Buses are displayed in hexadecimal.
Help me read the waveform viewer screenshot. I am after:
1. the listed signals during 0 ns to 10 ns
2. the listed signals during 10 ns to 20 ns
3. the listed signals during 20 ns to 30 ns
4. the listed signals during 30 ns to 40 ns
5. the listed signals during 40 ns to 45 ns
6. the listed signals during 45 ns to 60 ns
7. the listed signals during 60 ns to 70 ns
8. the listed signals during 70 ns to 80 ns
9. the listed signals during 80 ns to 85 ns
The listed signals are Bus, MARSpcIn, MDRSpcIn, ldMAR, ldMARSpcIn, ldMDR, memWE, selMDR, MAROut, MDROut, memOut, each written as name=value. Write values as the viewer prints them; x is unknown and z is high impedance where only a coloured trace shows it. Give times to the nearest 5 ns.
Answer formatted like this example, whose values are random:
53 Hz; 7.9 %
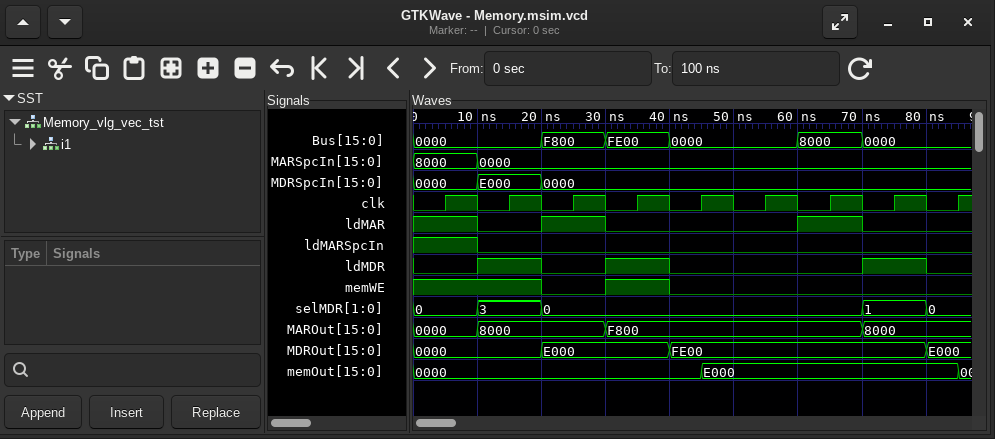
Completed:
Bus=0000, MARSpcIn=8000, MDRSpcIn=0000, ldMAR=1, ldMARSpcIn=1, ldMDR=0, memWE=1, selMDR=0, MAROut=0000, MDROut=0000, memOut=0000; Bus=0000, MARSpcIn=0000, MDRSpcIn=E000, ldMAR=0, ldMARSpcIn=0, ldMDR=1, memWE=1, selMDR=3, MAROut=8000, MDROut=0000, memOut=0000; Bus=F800, MARSpcIn=0000, MDRSpcIn=0000, ldMAR=1, ldMARSpcIn=0, ldMDR=0, memWE=0, selMDR=0, MAROut=8000, MDROut=E000, memOut=0000; Bus=FE00, MARSpcIn=0000, MDRSpcIn=0000, ldMAR=0, ldMARSpcIn=0, ldMDR=1, memWE=1, selMDR=0, MAROut=F800, MDROut=E000, memOut=0000; Bus=0000, MARSpcIn=0000, MDRSpcIn=0000, ldMAR=0, ldMARSpcIn=0, ldMDR=0, memWE=0, selMDR=0, MAROut=F800, MDROut=FE00, memOut=0000; Bus=0000, MARSpcIn=0000, MDRSpcIn=0000, ldMAR=0, ldMARSpcIn=0, ldMDR=0, memWE=0, selMDR=0, MAROut=F800, MDROut=FE00, memOut=E000; Bus=8000, MARSpcIn=0000, MDRSpcIn=0000, ldMAR=1, ldMARSpcIn=0, ldMDR=0, memWE=0, selMDR=0, MAROut=F800, MDROut=FE00, memOut=E000; Bus=0000, MARSpcIn=0000, MDRSpcIn=0000, ldMAR=0, ldMARSpcIn=0, ldMDR=1, memWE=0, selMDR=1, MAROut=8000, MDROut=FE00, memOut=E000; Bus=0000, MARSpcIn=0000, MDRSpcIn=0000, ldMAR=0, ldMARSpcIn=0, ldMDR=0, memWE=0, selMDR=0, MAROut=8000, MDROut=E000, memOut=E000
